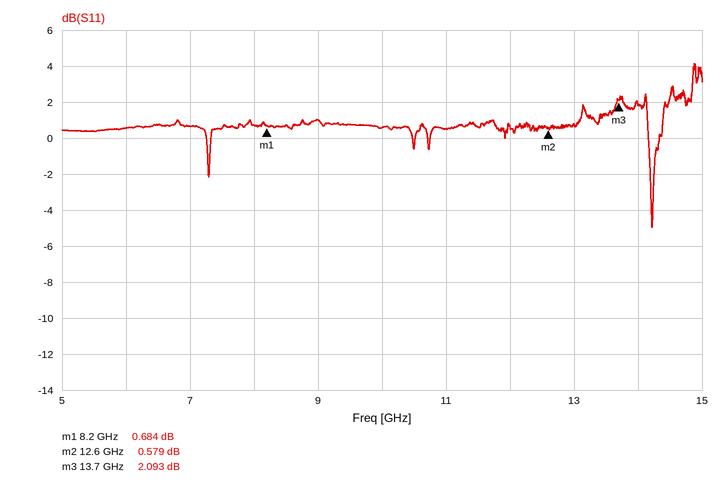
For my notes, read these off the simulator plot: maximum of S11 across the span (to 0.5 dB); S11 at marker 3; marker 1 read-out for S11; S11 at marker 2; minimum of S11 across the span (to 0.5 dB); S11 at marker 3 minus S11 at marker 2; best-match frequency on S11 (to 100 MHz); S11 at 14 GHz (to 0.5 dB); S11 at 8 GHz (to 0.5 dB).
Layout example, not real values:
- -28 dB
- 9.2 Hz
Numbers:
- 4.0 dB
- 2.093 dB
- 0.684 dB
- 0.579 dB
- -5.0 dB
- 1.514 dB
- 14.2 GHz
- 2.0 dB
- 0.5 dB
